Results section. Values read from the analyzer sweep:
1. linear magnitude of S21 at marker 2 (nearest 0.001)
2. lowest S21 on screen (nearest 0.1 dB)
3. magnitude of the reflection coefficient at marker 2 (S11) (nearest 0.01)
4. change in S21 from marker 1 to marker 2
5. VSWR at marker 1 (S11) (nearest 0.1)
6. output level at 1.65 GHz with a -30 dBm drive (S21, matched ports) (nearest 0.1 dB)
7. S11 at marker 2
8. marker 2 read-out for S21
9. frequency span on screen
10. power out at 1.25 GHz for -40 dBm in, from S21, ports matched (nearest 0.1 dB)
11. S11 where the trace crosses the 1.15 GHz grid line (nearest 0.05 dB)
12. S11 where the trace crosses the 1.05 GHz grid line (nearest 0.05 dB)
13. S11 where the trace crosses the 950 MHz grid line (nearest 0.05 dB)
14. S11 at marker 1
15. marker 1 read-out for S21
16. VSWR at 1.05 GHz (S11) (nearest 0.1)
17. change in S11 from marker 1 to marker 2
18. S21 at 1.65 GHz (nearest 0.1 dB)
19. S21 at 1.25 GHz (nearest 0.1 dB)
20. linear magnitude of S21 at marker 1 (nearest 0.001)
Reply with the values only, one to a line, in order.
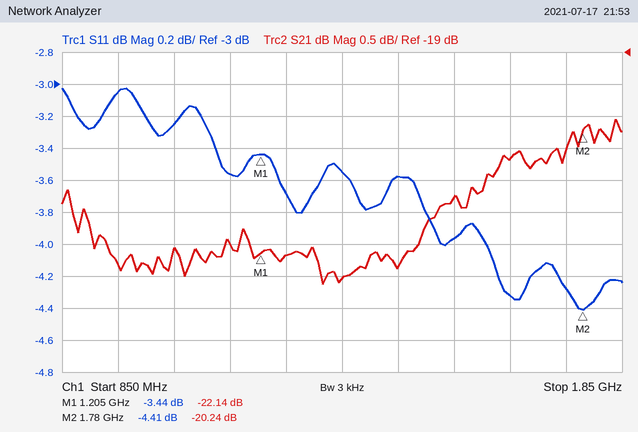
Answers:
0.097
-22.6 dB
0.60
1.90 dB
5.1
-50.7 dBm
-4.41 dB
-20.24 dB
1 GHz
-62.2 dBm
-3.55 dB
-3.25 dB
-3.05 dB
-3.44 dB
-22.14 dB
5.4
-0.97 dB
-20.7 dB
-22.2 dB
0.078
